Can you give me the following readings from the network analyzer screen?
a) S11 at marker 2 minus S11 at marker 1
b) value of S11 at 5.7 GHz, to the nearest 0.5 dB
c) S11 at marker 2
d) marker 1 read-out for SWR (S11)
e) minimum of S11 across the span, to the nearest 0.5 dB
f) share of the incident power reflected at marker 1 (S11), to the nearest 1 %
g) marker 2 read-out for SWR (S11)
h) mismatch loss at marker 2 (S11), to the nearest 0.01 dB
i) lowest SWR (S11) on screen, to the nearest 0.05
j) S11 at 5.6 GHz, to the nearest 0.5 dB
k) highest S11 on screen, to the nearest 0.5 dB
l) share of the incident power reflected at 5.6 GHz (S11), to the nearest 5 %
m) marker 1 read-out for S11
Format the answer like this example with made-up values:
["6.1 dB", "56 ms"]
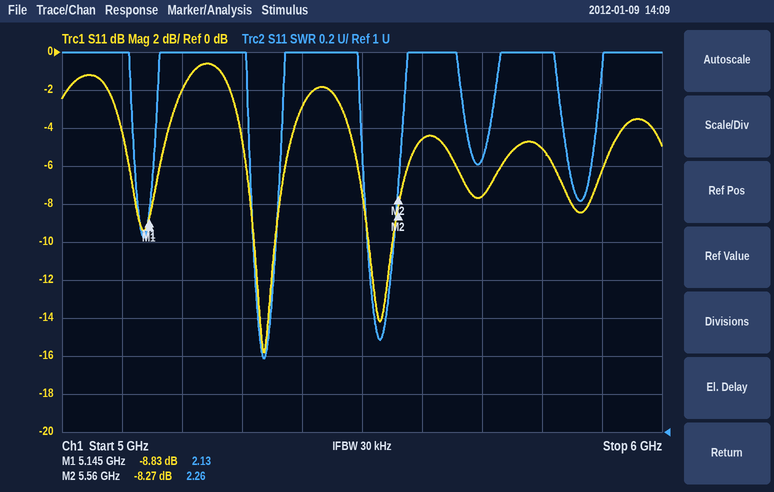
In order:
["0.56 dB", "-7.5 dB", "-8.27 dB", "2.13", "-16.0 dB", "13 %", "2.26", "0.70 dB", "1.40", "-4.5 dB", "-0.5 dB", "35 %", "-8.83 dB"]
